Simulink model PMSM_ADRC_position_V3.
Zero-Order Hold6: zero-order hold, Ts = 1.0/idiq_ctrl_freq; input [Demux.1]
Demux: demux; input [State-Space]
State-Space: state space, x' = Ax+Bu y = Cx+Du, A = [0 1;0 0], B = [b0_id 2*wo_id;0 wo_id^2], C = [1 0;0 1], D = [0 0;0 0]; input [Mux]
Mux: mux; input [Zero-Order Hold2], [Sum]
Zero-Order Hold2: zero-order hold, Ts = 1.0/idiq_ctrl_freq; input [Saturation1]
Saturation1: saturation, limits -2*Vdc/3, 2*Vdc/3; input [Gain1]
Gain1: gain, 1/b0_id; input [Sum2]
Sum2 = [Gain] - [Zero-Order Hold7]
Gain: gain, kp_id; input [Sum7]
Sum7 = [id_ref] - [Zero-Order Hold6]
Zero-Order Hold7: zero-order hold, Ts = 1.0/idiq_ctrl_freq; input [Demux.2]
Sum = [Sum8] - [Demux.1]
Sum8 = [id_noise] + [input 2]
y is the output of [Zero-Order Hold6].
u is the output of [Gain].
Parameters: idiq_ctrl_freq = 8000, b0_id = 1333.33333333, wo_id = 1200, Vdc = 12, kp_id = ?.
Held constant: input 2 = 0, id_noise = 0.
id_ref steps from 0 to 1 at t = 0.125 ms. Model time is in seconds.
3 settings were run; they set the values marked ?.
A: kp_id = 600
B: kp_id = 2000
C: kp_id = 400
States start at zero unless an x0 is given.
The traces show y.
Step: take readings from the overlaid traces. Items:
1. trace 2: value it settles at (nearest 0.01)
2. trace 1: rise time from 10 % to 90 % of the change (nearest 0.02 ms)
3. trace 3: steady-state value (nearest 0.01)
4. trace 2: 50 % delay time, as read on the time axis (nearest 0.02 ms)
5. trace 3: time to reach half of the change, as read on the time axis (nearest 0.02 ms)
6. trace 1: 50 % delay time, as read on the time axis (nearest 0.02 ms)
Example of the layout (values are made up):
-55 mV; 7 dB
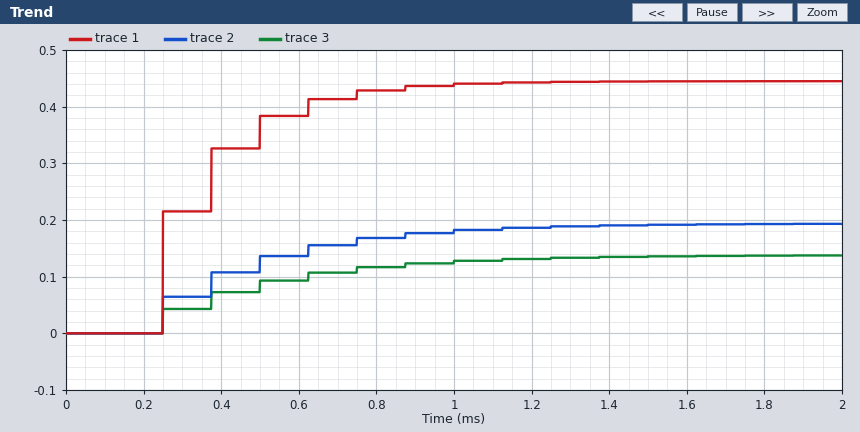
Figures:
0.19; 0.38 ms; 0.14; 0.38 ms; 0.38 ms; 0.38 ms
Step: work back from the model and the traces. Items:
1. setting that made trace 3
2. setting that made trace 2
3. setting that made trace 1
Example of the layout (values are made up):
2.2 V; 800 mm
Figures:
C; A; B
